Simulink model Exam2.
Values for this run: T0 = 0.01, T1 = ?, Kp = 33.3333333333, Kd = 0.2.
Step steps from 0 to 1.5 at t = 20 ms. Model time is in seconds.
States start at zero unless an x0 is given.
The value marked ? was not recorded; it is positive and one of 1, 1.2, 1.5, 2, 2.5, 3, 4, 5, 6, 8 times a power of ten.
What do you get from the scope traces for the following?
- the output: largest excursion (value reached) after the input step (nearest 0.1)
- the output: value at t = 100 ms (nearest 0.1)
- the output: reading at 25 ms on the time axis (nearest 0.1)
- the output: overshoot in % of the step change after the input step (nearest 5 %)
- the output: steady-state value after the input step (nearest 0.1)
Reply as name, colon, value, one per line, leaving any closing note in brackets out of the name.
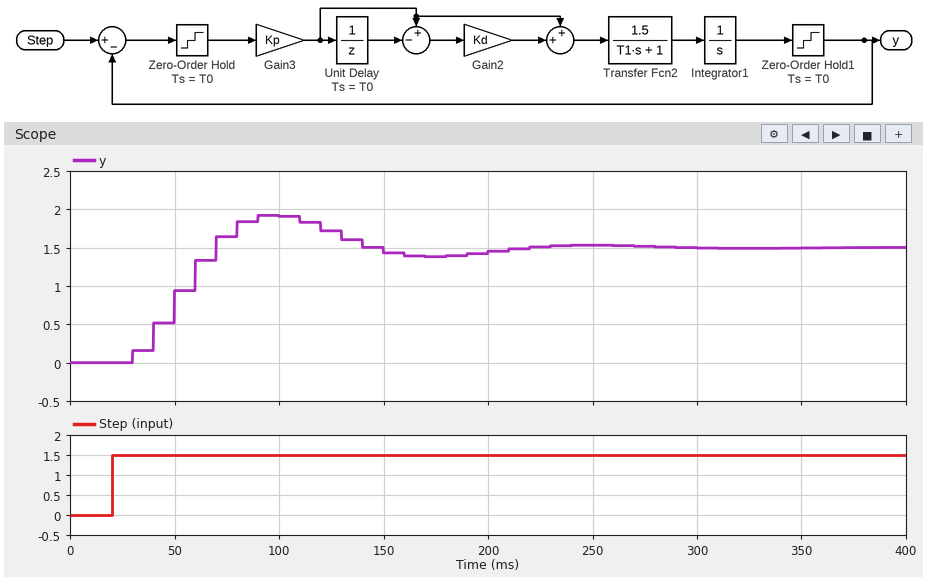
the output: largest excursion (value reached) after the input step: 1.9
the output: value at t = 100 ms: 1.9
the output: reading at 25 ms on the time axis: 0.0
the output: overshoot in % of the step change after the input step: 30 %
the output: steady-state value after the input step: 1.5
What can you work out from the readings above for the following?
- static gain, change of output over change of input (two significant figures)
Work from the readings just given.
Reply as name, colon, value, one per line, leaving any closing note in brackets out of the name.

static gain, change of output over change of input: 1.0
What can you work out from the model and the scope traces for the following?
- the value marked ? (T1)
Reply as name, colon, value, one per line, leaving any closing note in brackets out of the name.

the value marked ?: 0.025
